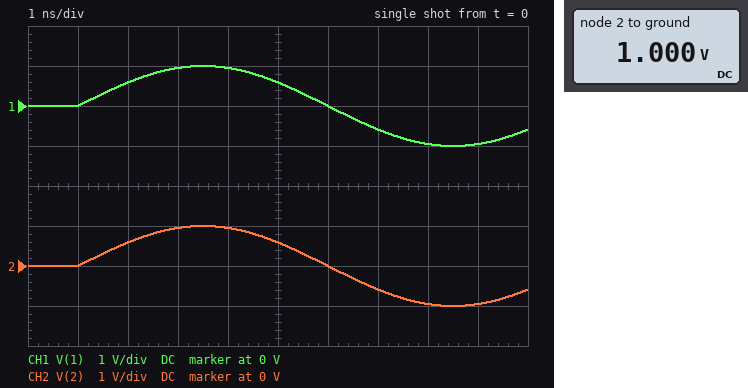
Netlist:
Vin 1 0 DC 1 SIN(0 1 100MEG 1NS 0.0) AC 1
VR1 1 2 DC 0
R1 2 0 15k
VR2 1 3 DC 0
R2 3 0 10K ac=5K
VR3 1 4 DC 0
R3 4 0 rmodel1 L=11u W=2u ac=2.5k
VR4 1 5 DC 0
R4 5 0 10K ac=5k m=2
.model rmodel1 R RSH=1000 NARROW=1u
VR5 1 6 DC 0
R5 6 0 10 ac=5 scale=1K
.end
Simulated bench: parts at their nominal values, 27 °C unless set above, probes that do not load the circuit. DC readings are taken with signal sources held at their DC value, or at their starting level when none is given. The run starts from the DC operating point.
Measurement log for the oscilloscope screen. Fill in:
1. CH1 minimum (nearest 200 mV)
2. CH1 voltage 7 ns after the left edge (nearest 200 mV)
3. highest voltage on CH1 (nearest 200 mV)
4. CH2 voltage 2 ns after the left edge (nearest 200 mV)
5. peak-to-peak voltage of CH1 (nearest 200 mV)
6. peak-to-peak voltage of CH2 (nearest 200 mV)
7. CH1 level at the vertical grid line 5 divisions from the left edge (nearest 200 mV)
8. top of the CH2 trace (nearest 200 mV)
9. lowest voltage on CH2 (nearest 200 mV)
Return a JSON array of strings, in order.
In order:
["-1.0 V", "-600 mV", "1.0 V", "600 mV", "2.0 V", "2.0 V", "600 mV", "1.0 V", "-1.0 V"]
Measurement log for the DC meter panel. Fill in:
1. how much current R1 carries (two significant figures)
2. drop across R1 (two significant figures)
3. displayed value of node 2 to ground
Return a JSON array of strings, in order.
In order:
["67 µA", "1.0 V", "1.000 V"]
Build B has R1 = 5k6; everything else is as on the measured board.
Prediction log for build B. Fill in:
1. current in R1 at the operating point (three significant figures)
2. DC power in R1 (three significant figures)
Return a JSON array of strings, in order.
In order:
["179 µA", "179 µW"]
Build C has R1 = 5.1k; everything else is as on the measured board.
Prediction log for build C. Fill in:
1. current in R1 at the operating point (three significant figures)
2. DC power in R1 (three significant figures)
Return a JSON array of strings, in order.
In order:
["196 µA", "196 µW"]
